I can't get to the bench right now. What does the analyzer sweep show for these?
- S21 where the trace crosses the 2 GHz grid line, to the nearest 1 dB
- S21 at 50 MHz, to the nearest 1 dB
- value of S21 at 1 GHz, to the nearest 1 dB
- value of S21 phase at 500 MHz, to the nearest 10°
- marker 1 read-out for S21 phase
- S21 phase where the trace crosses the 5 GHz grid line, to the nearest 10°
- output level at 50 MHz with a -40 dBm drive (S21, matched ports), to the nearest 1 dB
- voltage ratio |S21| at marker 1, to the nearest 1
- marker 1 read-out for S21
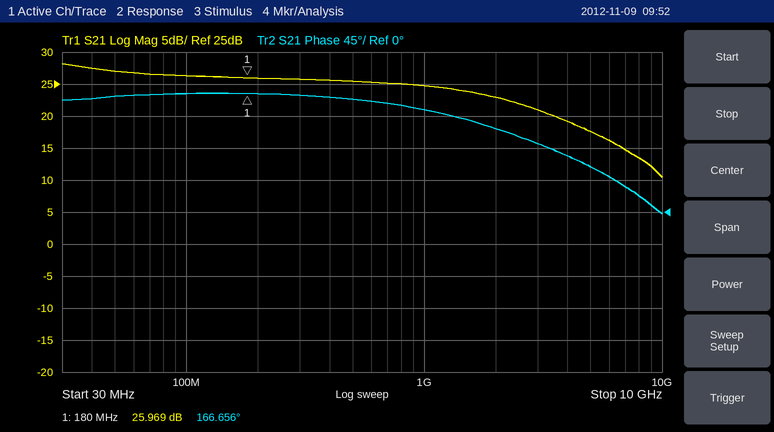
23 dB
27 dB
25 dB
160°
166.656°
60°
-13 dBm
20
25.969 dB
